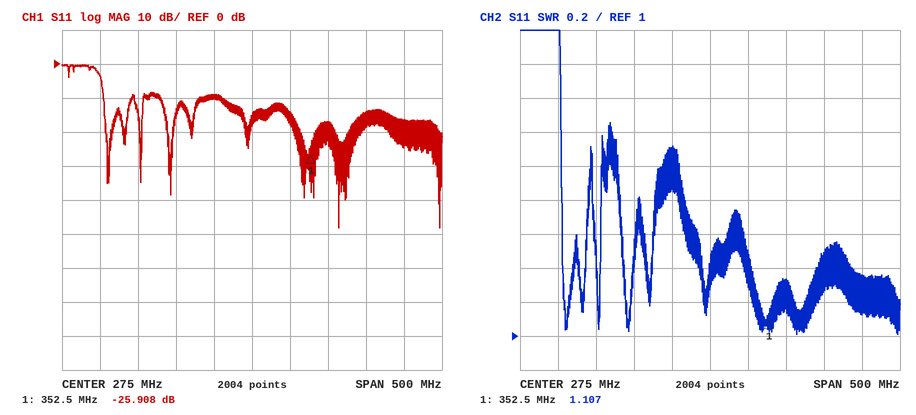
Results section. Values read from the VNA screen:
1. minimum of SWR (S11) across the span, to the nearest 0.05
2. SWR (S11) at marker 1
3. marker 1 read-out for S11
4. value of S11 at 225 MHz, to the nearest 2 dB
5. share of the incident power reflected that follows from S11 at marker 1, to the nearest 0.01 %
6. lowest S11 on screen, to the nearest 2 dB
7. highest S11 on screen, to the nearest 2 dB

1.00
1.107
-25.908 dB
-10 dB
0.26 %
-48 dB
0 dB
